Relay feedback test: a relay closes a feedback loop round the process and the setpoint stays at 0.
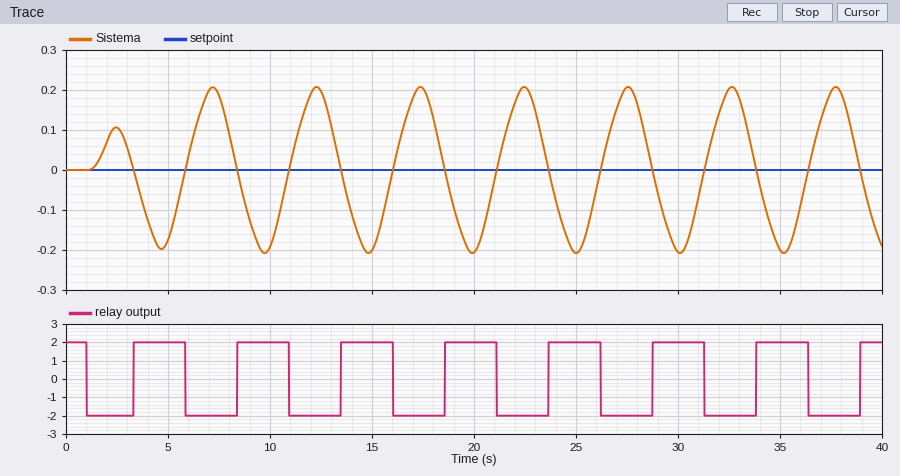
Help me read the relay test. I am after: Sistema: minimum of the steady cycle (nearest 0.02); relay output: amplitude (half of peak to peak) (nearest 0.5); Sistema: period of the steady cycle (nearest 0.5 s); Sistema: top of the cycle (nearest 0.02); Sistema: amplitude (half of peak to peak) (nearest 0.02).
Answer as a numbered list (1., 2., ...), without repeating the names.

1. -0.20
2. 2.0
3. 5.0 s
4. 0.20
5. 0.20
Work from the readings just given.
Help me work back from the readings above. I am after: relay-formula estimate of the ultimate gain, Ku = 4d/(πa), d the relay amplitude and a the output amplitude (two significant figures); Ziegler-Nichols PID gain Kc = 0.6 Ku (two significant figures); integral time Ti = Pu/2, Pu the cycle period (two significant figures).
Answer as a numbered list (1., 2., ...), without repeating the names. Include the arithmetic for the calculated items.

1. 4 × 2 / (π × 0.2) = 13
2. 0.6 × 13 = 7.8
3. 5 / 2 = 2.5 s
